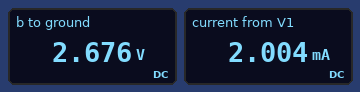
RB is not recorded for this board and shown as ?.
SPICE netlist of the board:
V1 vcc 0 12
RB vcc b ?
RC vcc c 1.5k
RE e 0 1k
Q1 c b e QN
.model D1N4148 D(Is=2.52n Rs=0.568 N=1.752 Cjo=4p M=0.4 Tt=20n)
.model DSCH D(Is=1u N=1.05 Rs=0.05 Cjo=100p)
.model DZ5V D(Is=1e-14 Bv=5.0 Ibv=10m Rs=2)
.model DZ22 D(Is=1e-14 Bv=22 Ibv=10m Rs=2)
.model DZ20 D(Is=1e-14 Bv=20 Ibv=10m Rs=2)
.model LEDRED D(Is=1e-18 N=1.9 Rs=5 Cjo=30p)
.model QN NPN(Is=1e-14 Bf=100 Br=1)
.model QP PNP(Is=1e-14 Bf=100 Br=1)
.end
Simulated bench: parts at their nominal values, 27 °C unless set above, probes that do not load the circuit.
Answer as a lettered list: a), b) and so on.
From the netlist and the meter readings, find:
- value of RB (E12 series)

a) 470 kΩ
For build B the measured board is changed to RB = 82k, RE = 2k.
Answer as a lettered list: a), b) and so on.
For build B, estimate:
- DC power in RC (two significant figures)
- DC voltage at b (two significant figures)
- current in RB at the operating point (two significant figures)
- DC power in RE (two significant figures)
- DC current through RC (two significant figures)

a) 17 mW
b) 7.5 V
c) 55 µA
d) 23 mW
e) 3.4 mA
